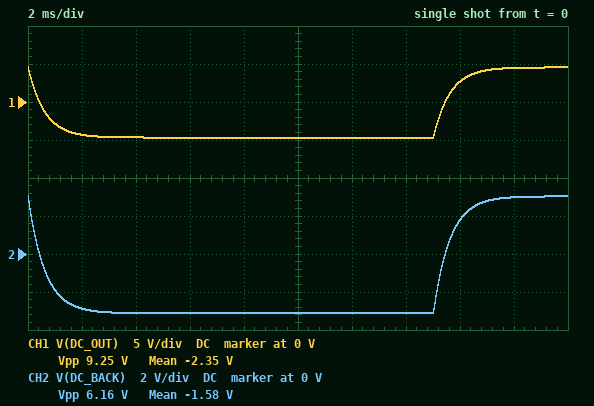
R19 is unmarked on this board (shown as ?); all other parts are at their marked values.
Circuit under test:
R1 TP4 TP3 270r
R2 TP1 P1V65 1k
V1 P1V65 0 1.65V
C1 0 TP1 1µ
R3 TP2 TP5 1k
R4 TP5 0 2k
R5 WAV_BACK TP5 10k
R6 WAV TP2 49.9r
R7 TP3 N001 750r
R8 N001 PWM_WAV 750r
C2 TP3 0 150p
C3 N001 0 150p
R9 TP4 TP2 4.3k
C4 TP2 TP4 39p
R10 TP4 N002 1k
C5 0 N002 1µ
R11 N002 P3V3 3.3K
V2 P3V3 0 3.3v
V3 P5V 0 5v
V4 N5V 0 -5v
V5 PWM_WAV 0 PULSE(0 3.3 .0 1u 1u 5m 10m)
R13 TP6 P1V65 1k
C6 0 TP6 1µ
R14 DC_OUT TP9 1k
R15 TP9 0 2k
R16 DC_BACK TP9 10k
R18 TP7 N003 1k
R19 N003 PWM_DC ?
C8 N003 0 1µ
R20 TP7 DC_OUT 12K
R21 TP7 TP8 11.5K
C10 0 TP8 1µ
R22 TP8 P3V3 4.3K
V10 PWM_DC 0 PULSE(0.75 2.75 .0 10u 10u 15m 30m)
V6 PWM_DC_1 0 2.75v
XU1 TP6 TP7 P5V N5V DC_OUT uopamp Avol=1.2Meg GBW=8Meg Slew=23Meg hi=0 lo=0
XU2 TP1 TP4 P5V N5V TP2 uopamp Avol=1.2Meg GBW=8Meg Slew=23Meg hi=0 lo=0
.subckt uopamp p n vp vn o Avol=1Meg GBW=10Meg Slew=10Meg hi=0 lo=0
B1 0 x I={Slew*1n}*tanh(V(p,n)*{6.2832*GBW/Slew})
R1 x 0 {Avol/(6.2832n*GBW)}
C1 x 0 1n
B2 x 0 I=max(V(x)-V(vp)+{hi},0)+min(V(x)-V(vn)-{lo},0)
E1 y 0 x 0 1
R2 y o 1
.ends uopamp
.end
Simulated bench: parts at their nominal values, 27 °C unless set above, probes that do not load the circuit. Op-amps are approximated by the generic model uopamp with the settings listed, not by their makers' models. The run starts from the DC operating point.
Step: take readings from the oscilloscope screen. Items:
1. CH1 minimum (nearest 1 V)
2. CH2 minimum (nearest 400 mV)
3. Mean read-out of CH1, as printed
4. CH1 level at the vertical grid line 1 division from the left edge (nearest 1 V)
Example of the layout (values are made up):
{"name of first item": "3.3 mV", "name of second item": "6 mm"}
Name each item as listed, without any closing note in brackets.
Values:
{"CH1 minimum": "-5 V", "CH2 minimum": "-3.2 V", "Mean read-out of CH1, as printed": "-2.35 V", "CH1 level at the vertical grid line 1 division from the left edge": "-4 V"}
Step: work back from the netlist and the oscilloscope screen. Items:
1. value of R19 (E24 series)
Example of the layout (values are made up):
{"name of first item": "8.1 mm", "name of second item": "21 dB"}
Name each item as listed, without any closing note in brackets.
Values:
{"value of R19": "1.6 kΩ"}
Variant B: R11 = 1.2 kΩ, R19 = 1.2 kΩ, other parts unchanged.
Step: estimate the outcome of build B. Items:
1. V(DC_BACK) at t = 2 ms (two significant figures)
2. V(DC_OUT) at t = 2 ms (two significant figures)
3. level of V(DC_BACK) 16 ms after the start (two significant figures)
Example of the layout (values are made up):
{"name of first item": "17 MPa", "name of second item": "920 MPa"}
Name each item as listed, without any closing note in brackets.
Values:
{"V(DC_BACK) at t = 2 ms": "-3.3 V", "V(DC_OUT) at t = 2 ms": "-5.0 V", "level of V(DC_BACK) 16 ms after the start": "2.3 V"}
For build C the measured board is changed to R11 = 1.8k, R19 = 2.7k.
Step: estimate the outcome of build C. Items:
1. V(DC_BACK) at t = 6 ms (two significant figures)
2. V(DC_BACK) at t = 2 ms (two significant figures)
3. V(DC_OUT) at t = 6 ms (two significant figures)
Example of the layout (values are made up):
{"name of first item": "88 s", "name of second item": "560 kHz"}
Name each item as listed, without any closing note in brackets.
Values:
{"V(DC_BACK) at t = 6 ms": "-2.1 V", "V(DC_BACK) at t = 2 ms": "-1.8 V", "V(DC_OUT) at t = 6 ms": "-3.2 V"}
